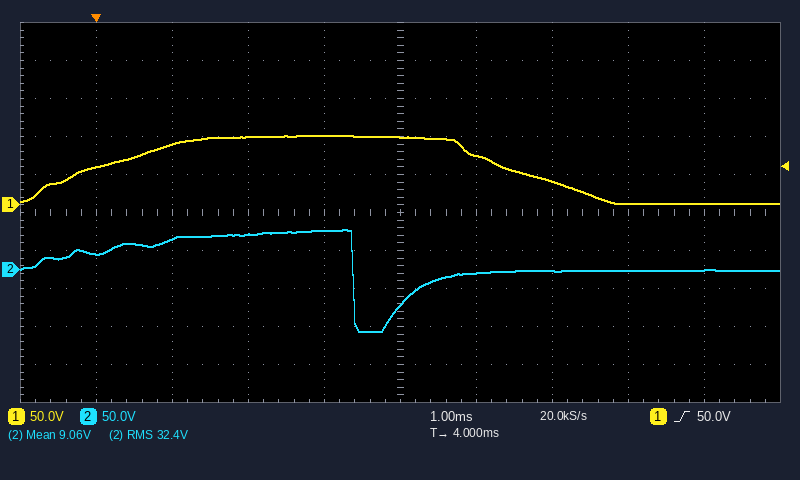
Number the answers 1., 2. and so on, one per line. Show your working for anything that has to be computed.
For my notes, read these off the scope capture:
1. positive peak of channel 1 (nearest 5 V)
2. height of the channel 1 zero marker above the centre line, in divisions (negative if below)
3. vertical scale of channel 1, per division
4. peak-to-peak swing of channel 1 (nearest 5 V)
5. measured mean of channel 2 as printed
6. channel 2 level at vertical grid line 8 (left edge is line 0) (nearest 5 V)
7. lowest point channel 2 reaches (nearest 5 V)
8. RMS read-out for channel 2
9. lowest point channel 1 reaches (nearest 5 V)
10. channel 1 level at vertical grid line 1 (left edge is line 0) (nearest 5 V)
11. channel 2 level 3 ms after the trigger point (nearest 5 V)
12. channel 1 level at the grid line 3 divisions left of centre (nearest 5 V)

1. 90 V
2. +0.2 div
3. 50 V
4. 90 V − (0 V) = 90 V
5. 9.06 V
6. 0 V
7. -80 V
8. 32.4 V
9. 0 V
10. 50 V
11. 50 V
12. 80 V
